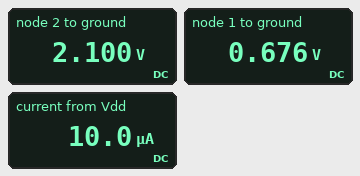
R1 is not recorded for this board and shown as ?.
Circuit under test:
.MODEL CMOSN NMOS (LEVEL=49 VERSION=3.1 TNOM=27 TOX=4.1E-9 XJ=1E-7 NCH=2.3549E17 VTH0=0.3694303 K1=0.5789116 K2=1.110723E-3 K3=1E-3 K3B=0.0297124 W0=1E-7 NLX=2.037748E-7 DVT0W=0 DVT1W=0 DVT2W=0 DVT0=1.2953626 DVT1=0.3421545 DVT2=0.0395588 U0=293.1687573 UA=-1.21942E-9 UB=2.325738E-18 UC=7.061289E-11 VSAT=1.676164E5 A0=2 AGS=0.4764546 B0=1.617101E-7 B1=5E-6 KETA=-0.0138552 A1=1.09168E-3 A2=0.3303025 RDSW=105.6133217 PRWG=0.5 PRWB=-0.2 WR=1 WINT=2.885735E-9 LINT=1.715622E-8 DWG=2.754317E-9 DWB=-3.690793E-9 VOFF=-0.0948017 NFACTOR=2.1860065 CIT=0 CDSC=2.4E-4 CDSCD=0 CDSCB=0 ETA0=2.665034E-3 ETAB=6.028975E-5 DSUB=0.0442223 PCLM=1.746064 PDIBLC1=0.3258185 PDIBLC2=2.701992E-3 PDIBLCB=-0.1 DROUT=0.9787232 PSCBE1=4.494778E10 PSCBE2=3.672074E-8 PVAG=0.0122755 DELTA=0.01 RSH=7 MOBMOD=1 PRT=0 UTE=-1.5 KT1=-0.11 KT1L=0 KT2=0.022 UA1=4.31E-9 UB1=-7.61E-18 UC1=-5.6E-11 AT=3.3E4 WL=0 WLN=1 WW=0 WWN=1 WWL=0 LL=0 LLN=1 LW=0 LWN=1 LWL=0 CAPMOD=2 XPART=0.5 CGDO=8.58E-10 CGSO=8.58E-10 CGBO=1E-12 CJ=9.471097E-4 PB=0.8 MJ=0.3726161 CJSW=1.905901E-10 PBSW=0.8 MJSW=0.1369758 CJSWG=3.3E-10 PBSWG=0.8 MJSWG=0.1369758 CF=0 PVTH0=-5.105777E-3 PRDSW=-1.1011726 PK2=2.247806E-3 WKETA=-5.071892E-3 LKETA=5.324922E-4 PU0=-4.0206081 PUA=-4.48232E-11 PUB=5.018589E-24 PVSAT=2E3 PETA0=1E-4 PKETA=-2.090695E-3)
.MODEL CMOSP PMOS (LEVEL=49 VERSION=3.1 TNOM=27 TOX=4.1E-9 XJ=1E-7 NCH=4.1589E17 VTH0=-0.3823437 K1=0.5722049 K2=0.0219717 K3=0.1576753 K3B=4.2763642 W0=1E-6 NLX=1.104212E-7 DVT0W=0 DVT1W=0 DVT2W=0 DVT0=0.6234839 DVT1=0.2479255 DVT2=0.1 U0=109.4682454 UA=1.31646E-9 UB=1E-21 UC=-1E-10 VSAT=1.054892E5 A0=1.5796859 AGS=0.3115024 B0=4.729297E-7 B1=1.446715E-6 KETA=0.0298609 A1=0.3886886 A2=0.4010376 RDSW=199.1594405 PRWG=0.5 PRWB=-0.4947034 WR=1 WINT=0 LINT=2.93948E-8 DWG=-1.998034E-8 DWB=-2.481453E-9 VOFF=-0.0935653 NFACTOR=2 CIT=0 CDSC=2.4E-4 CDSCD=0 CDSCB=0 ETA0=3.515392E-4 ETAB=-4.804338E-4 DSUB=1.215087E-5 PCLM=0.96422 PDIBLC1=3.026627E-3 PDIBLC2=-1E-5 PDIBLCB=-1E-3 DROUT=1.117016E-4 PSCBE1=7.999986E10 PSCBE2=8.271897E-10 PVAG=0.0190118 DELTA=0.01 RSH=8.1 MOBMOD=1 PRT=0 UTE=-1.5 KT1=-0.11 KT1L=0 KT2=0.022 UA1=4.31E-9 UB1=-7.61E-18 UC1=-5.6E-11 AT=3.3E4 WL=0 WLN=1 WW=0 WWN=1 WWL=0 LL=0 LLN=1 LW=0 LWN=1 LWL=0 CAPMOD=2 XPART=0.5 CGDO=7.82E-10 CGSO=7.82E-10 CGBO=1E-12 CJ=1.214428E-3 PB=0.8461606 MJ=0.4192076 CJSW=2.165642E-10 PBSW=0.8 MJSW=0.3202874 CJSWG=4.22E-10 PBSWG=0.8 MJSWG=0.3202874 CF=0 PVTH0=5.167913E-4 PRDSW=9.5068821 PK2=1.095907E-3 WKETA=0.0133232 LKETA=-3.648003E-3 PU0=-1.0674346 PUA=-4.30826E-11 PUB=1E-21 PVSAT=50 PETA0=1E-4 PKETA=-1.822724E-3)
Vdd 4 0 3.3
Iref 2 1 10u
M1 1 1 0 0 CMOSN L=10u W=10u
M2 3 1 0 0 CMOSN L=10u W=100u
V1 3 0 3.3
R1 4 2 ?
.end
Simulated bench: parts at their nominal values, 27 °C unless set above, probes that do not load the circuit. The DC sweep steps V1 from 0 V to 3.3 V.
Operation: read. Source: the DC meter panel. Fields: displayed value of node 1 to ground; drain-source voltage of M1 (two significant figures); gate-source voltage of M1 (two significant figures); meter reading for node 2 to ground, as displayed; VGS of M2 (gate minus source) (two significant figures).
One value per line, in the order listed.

0.676 V
680 mV
680 mV
2.100 V
680 mV
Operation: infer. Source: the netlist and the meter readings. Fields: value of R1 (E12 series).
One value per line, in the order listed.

120 kΩ
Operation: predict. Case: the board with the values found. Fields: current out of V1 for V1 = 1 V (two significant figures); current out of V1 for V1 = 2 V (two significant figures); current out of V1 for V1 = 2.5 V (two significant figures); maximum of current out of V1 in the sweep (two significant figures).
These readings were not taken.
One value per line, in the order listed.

100 µA
100 µA
100 µA
100 µA
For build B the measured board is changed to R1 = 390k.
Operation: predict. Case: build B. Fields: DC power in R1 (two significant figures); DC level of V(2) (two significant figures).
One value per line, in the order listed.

39 µW
-600 mV
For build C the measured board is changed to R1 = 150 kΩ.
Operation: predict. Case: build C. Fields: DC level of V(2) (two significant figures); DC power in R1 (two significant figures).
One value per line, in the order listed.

1.8 V
15 µW
